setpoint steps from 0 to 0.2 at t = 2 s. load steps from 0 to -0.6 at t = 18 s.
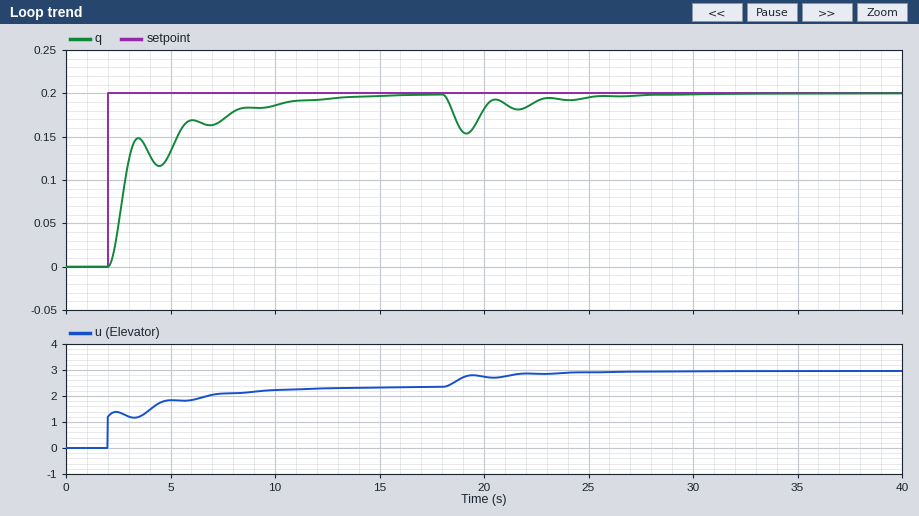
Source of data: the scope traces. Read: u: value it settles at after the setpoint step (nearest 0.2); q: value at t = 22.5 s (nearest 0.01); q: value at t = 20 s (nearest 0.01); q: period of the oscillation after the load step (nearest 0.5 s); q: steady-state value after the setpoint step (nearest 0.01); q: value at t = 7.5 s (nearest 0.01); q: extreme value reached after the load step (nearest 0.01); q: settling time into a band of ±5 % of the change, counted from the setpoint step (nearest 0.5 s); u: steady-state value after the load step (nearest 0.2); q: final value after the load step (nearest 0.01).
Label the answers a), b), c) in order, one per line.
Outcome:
a) 2.4
b) 0.19
c) 0.18
d) 2.5 s
e) 0.20
f) 0.17
g) 0.15
h) 8.5 s
i) 3.0
j) 0.20
